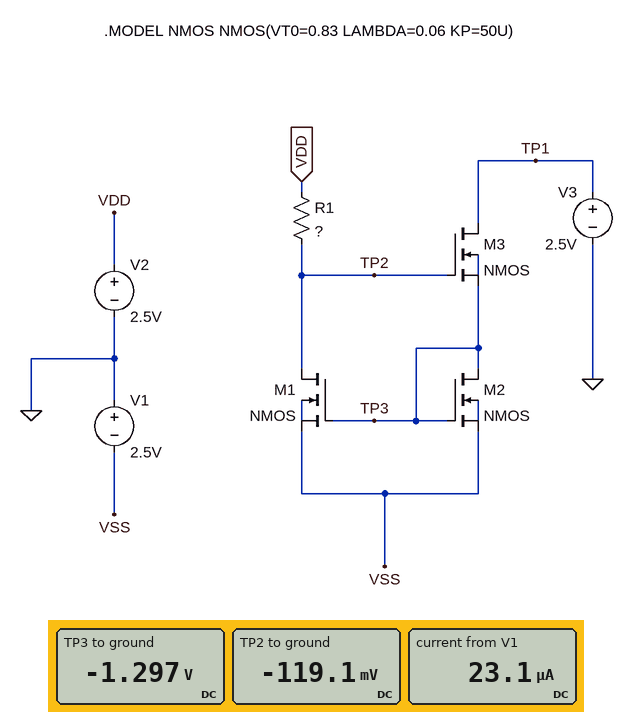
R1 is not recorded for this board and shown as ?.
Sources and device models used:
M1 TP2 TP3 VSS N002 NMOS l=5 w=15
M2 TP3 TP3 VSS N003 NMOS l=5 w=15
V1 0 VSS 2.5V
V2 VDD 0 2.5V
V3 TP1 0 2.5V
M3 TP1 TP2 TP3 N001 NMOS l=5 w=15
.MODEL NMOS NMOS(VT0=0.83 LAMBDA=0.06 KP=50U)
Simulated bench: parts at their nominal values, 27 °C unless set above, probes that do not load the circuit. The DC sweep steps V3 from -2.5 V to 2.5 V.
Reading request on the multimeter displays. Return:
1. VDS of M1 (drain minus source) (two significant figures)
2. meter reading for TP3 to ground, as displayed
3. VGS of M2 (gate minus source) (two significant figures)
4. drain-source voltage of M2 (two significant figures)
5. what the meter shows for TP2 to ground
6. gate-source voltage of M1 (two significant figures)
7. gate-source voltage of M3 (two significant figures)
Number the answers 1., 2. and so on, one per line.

1. 2.4 V
2. -1.297 V
3. 1.2 V
4. 1.2 V
5. -119.1 mV
6. 1.2 V
7. 1.2 V
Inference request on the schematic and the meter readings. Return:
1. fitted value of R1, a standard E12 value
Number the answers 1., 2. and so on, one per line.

1. 220 kΩ
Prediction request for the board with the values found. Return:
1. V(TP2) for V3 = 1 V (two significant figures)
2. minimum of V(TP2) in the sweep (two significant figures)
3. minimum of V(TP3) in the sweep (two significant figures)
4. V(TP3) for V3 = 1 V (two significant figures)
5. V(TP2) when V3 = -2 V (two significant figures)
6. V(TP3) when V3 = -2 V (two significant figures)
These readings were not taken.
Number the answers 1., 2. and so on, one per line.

1. -110 mV
2. -120 mV
3. -2.5 V
4. -1.3 V
5. 2.5 V
6. -2.0 V
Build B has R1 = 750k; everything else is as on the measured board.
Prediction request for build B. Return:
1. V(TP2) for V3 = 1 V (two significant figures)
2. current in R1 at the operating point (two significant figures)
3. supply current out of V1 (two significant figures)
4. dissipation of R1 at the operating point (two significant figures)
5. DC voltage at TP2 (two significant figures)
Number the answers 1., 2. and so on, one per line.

1. -420 mV
2. 3.9 µA
3. 7.6 µA
4. 11 µW
5. -430 mV
